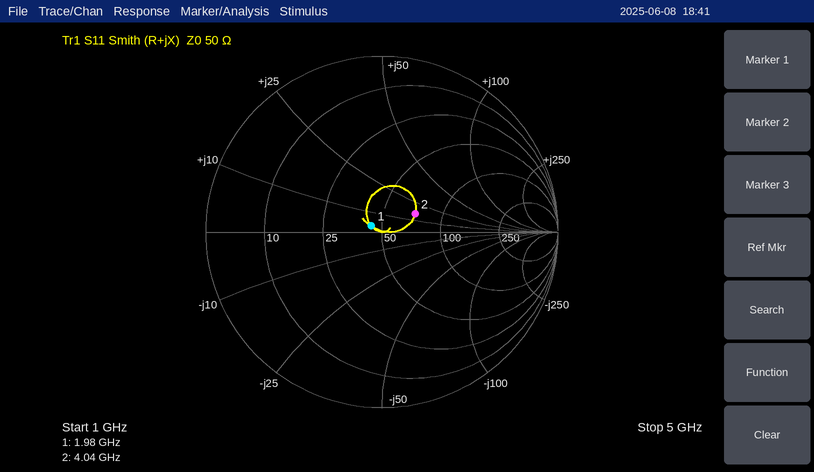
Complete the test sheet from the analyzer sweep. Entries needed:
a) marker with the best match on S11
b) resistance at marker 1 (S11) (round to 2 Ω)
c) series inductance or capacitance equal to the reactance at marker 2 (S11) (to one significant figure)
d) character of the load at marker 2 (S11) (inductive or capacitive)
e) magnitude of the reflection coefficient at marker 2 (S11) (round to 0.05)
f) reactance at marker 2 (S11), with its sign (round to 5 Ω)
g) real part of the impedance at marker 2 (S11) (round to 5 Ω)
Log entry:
marker 1
44 Ω
600 pH
inductive
0.20
+15 Ω
70 Ω
